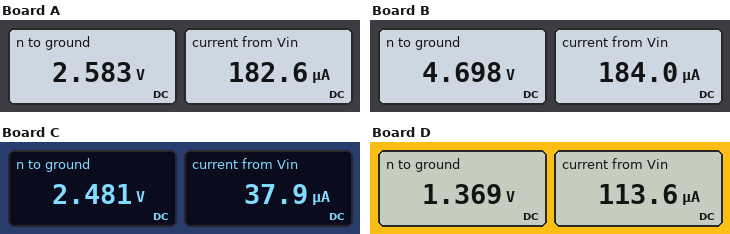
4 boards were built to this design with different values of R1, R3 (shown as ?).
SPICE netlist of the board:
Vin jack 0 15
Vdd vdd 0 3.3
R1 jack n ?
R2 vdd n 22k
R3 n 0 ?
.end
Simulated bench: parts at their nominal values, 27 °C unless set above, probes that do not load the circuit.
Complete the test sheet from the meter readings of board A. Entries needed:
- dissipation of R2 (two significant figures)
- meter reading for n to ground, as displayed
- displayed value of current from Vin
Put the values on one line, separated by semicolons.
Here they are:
23 µW; 2.583 V; 182.6 µA
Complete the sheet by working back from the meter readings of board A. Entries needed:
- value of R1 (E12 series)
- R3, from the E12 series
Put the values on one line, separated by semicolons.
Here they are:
68 kΩ; 12 kΩ
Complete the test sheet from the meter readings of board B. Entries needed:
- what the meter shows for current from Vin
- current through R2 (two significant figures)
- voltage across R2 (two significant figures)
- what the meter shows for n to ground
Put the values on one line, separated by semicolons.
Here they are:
184.0 µA; 64 µA; 1.4 V; 4.698 V
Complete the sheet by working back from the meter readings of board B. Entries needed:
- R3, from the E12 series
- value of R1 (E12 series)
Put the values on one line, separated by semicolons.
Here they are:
39 kΩ; 56 kΩ
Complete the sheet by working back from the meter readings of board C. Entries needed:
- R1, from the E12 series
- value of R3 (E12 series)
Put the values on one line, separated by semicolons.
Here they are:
330 kΩ; 33 kΩ
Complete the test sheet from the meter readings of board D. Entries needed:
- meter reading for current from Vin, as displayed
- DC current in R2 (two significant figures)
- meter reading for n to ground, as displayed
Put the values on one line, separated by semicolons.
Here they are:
113.6 µA; 88 µA; 1.369 V
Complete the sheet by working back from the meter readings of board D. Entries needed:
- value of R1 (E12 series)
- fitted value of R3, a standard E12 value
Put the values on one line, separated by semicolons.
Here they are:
120 kΩ; 6.8 kΩ
